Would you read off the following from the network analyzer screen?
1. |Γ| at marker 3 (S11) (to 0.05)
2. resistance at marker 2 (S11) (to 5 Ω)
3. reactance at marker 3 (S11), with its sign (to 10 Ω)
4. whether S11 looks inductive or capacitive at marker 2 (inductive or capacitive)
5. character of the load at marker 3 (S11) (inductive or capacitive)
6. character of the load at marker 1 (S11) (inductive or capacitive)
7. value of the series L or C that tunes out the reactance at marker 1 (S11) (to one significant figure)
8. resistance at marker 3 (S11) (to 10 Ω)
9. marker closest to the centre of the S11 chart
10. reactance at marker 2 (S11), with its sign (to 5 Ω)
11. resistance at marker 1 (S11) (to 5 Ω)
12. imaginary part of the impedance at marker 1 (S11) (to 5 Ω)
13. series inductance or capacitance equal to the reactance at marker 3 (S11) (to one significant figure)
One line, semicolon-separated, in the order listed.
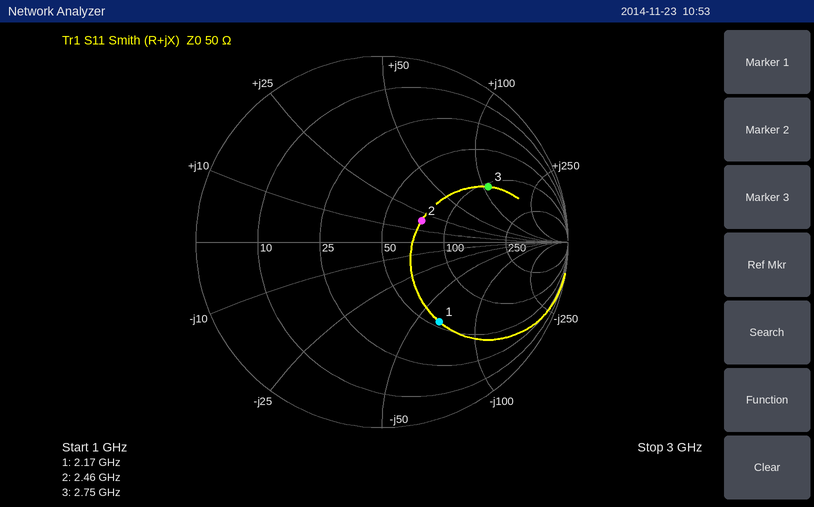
0.65; 75 Ω; +110 Ω; inductive; inductive; capacitive; 5 nH; 110 Ω; marker 2; +20 Ω; 55 Ω; -65 Ω; 6 nH
